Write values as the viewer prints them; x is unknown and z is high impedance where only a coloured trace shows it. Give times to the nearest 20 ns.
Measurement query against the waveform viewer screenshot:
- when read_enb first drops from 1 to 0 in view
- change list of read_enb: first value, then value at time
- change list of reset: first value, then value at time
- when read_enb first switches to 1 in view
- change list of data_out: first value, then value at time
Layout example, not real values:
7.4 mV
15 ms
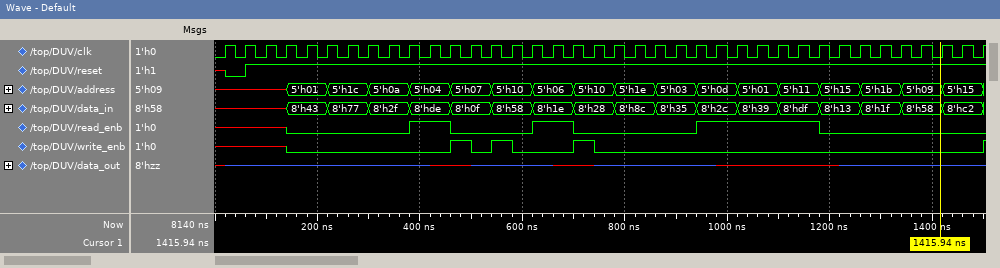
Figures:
460 ns
x, 0 at 140 ns, 1 at 380 ns, 0 at 460 ns, 1 at 620 ns, 0 at 700 ns, 1 at 940 ns, 0 at 1180 ns
x, 0 at 20 ns, 1 at 60 ns
380 ns
x, z at 20 ns, x at 420 ns, z at 500 ns, x at 660 ns, z at 740 ns, x at 980 ns, z at 1220 ns
